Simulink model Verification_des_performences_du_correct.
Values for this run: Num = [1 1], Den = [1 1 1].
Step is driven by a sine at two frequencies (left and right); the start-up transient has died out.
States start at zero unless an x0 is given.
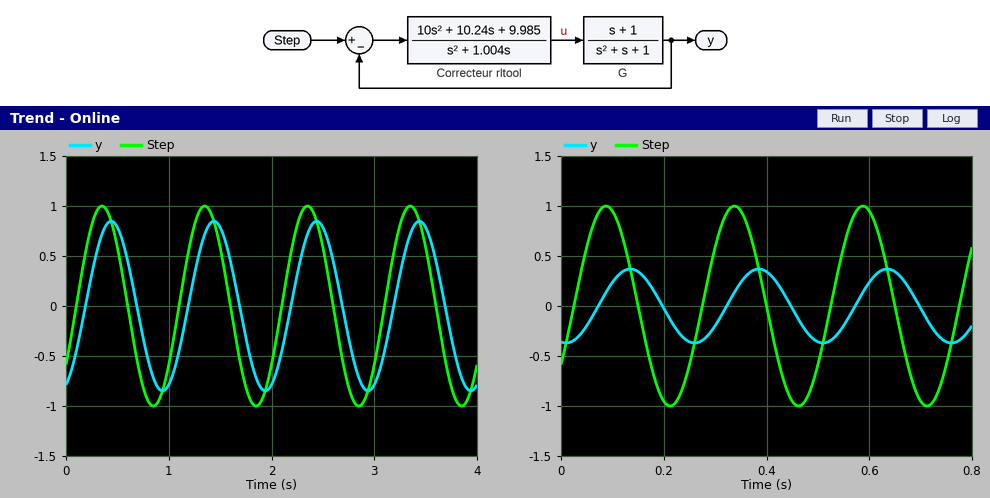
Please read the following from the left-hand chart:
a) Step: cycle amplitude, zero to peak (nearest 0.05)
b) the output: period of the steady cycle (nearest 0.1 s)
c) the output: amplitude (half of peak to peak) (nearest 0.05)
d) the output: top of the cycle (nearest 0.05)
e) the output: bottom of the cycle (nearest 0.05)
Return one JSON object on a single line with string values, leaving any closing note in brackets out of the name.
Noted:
{"Step: cycle amplitude, zero to peak": "1.00", "the output: period of the steady cycle": "1.0 s", "the output: amplitude (half of peak to peak)": "0.85", "the output: top of the cycle": "0.85", "the output: bottom of the cycle": "-0.85"}
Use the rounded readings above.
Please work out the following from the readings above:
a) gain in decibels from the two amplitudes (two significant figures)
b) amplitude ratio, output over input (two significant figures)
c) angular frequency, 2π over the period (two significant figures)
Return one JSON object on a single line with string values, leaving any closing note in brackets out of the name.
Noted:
{"gain in decibels from the two amplitudes": "-1.4 dB", "amplitude ratio, output over input": "0.85", "angular frequency, 2π over the period": "6.3 rad/s"}
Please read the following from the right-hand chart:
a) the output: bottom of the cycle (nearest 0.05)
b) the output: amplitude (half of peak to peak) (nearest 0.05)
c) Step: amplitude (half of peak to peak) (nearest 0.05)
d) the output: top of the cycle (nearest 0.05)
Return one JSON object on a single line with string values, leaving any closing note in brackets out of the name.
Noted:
{"the output: bottom of the cycle": "-0.35", "the output: amplitude (half of peak to peak)": "0.35", "Step: amplitude (half of peak to peak)": "1.00", "the output: top of the cycle": "0.35"}
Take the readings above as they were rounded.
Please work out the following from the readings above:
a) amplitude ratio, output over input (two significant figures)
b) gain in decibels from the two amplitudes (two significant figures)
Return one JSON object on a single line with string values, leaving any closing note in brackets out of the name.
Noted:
{"amplitude ratio, output over input": "0.35", "gain in decibels from the two amplitudes": "-9.1 dB"}
